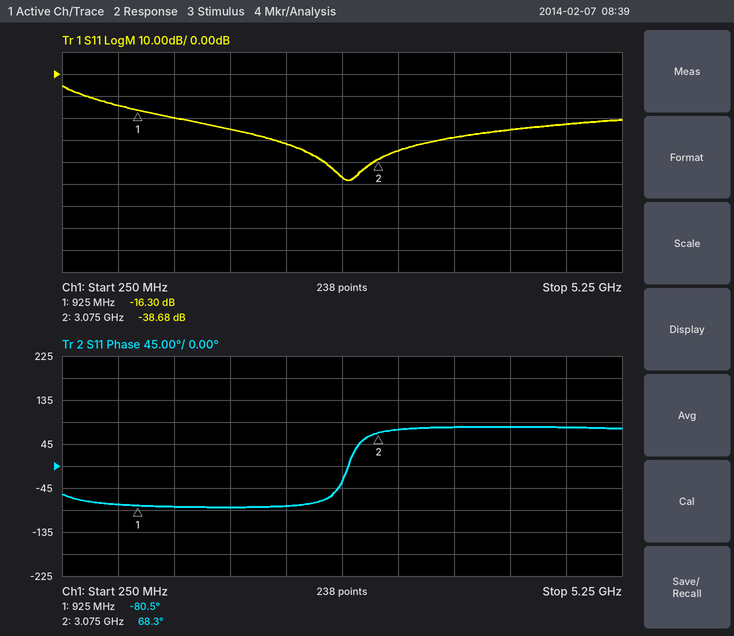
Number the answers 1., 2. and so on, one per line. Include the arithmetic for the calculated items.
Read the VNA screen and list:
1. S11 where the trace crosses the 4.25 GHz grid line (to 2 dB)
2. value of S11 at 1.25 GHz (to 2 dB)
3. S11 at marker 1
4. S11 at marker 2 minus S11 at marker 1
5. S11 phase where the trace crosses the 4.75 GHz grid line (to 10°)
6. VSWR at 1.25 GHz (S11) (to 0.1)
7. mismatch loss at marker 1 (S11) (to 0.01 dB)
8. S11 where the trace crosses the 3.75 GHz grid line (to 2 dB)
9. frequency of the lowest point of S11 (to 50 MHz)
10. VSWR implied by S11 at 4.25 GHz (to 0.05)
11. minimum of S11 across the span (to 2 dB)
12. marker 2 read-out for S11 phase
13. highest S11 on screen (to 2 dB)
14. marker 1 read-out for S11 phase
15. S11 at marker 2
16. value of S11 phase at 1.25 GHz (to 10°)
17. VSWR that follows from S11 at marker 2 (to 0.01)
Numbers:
1. -26 dB
2. -20 dB
3. -16.30 dB
4. -38.68 − (-16.3) = -22.38 dB
5. 80°
6. |Γ| = 10^(-20/20) = 0.1000; VSWR = (1 + 0.1000)/(1 − 0.1000) ≈ 1.2
7. −10 log10(1 − 10^(-16.3/10)) ≈ 0.10 dB
8. -28 dB
9. 2.80 GHz
10. |Γ| = 10^(-26/20) = 0.0501; VSWR = (1 + 0.0501)/(1 − 0.0501) ≈ 1.11, so 1.10 to the nearest 0.05
11. -48 dB
12. 68.3°
13. -6 dB
14. -80.5°
15. -38.68 dB
16. -80°
17. (1 + 0.0116)/(1 − 0.0116) ≈ 1.02
